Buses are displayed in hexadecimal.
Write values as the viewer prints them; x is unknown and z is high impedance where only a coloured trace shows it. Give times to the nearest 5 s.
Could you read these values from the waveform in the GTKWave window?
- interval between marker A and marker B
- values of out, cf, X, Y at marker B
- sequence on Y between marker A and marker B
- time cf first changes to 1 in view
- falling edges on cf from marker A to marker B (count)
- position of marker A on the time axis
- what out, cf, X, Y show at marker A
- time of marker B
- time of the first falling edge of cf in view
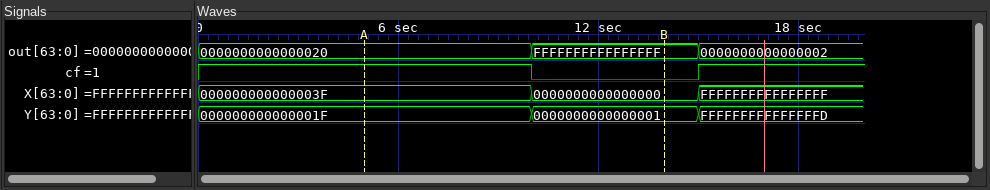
10 s
out=FFFFFFFFFFFFFFFF, cf=0, X=0000000000000000, Y=0000000000000001
000000000000001F, 0000000000000001
15 s
1
5 s
out=0000000000000020, cf=1, X=000000000000003F, Y=000000000000001F
15 s
10 s
